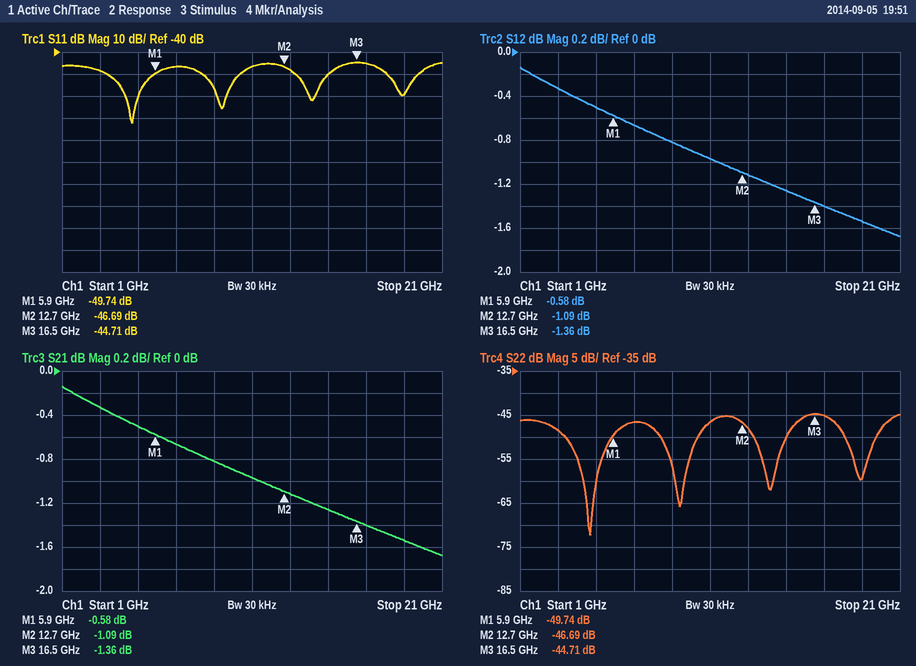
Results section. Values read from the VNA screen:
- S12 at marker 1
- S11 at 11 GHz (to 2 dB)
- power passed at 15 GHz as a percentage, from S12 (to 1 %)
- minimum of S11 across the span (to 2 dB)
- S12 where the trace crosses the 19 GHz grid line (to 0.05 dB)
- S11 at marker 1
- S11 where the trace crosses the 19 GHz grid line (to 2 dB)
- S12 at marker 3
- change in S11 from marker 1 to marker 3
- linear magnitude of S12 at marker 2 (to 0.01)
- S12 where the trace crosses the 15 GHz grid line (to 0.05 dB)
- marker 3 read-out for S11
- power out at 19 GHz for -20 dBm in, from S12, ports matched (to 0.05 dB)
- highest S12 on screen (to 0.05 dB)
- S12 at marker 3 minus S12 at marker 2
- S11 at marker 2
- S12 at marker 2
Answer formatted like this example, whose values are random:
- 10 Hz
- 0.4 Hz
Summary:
- -0.58 dB
- -46 dB
- 75 %
- -72 dB
- -1.55 dB
- -49.74 dB
- -60 dB
- -1.36 dB
- 5.03 dB
- 0.88
- -1.25 dB
- -44.71 dB
- -21.55 dBm
- -0.15 dB
- -0.27 dB
- -46.69 dB
- -1.09 dB
